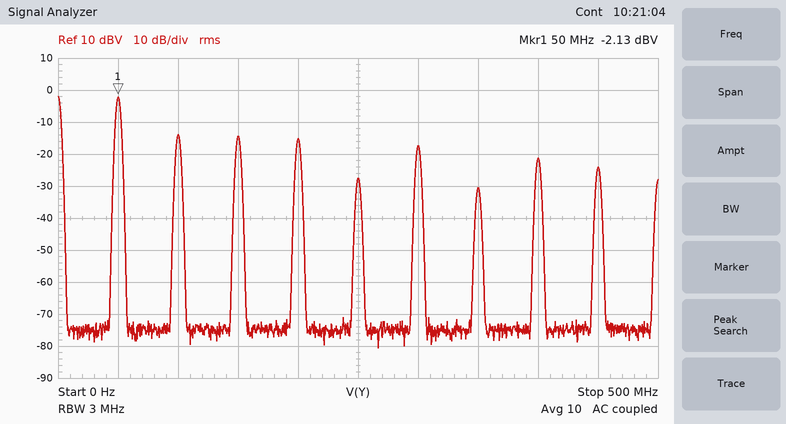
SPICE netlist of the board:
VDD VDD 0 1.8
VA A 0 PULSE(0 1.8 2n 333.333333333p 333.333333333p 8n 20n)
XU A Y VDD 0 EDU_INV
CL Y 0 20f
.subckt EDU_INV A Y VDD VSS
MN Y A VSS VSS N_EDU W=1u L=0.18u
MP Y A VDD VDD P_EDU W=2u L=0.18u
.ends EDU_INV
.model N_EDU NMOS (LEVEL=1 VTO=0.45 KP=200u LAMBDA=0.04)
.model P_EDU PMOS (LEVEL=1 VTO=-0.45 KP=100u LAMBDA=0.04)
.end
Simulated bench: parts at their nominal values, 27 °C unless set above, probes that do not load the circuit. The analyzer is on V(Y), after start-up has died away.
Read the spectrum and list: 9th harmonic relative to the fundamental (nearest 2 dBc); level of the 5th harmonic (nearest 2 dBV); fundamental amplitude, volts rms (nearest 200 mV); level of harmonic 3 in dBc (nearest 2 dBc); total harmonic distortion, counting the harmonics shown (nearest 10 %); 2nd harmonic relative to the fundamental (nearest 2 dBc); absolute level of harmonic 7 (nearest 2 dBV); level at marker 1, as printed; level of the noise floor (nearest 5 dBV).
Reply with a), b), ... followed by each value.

a) -22 dBc
b) -28 dBV
c) 800 mV
d) -12 dBc
e) 50 %
f) -12 dBc
g) -30 dBV
h) -2.13 dBV
i) -75 dBV
